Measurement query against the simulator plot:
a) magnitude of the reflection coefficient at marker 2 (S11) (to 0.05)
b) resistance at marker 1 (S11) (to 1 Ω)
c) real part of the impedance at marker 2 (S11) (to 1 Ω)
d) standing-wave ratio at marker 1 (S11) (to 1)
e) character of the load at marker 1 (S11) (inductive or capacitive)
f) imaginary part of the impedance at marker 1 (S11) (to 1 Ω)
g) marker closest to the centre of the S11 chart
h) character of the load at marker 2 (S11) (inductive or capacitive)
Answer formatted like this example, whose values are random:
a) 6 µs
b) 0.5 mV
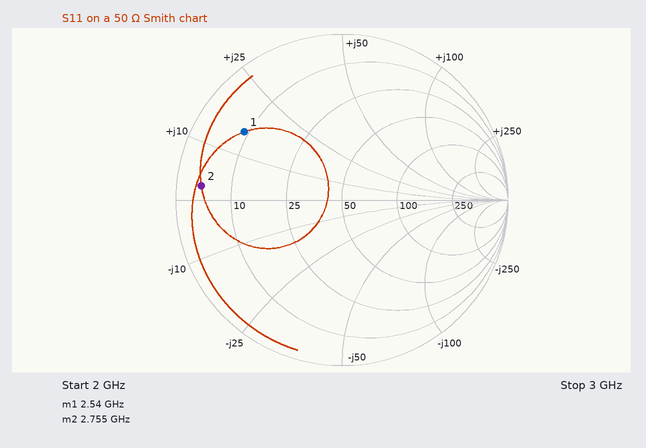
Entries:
a) 0.85
b) 9 Ω
c) 4 Ω
d) 6
e) inductive
f) +15 Ω
g) marker 1
h) inductive
